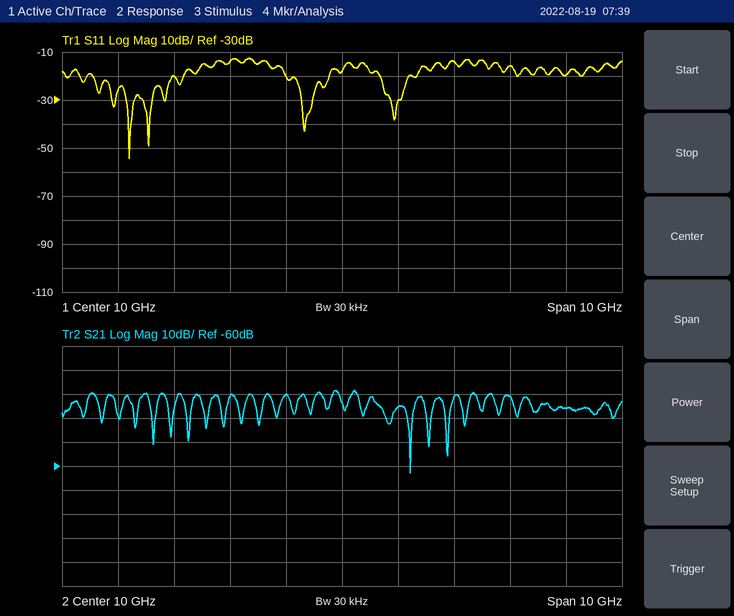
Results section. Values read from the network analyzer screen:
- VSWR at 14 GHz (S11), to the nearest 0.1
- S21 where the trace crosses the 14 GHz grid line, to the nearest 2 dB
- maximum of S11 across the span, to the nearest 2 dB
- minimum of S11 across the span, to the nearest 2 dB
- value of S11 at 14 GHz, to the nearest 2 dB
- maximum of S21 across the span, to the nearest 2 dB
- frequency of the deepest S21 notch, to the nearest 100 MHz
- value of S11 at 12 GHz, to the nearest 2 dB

1.2
-36 dB
-12 dB
-54 dB
-20 dB
-28 dB
11.2 GHz
-14 dB
